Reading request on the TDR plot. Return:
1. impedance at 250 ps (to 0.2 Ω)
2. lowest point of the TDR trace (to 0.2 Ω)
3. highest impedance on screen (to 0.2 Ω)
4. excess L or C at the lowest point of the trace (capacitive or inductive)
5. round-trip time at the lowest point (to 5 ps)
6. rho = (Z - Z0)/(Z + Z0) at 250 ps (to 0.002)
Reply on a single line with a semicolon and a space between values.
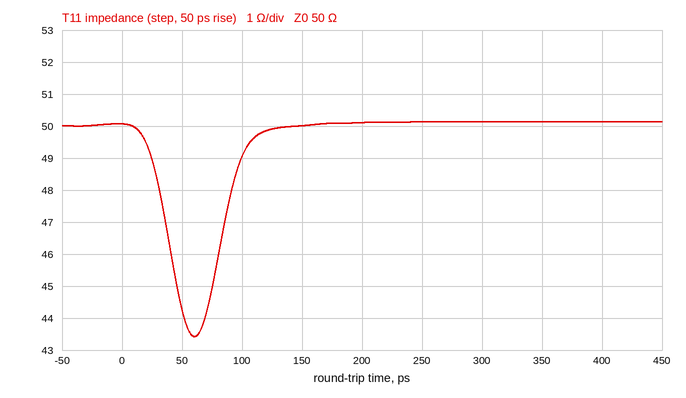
50.2 Ω; 43.4 Ω; 50.2 Ω; capacitive; 60 ps; +0.002
